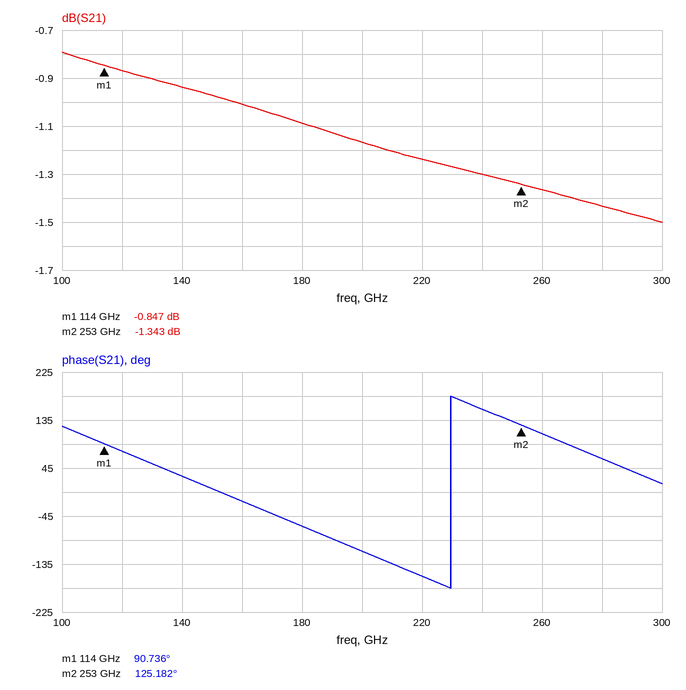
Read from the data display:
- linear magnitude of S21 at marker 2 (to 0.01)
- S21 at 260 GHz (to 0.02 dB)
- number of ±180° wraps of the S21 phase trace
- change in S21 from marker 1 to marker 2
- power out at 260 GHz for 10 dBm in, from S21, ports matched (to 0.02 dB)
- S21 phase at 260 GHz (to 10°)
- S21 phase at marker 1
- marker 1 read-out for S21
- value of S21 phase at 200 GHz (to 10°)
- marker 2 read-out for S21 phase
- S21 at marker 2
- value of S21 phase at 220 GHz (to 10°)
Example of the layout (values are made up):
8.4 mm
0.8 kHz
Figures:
0.86
-1.36 dB
1
-0.496 dB
8.64 dBm
110°
90.736°
-0.847 dB
-110°
125.182°
-1.343 dB
-160°
